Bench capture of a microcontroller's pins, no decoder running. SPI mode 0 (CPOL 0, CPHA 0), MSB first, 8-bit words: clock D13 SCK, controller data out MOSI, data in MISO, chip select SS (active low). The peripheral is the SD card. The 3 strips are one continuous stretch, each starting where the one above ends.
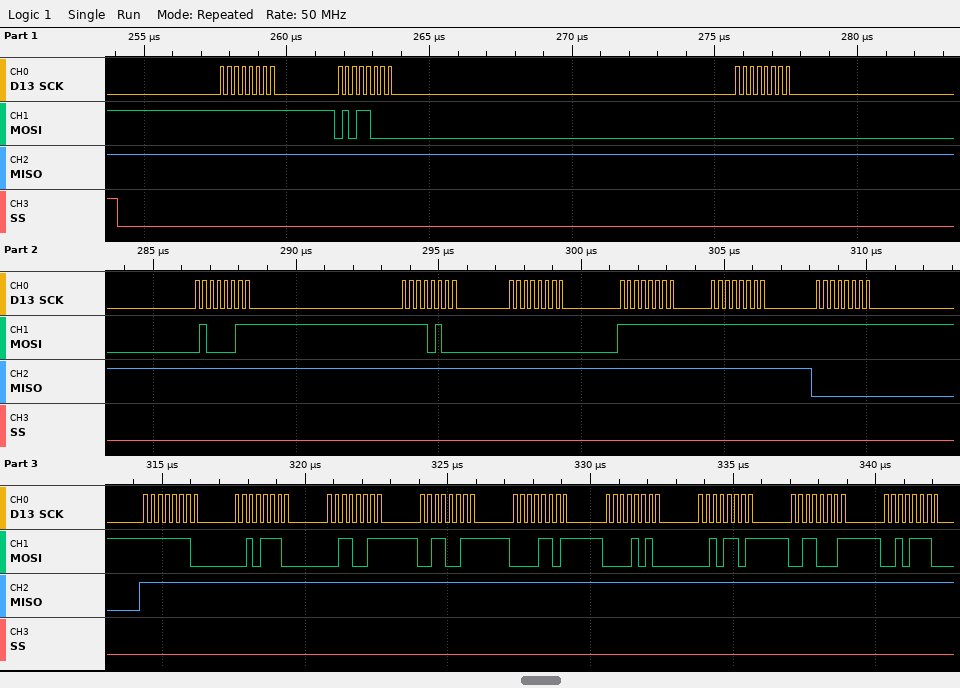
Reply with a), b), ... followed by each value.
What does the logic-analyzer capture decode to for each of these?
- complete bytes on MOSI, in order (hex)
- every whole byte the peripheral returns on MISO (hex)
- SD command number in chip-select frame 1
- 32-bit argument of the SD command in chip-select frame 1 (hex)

a) 0xFF 0x58 0x00 0x43 0xF4 0x00 0xFF 0xFF 0xFF 0xFE 0x2E 0x33 0x33 0x0D 0x0A 0x2D 0x31 0x2E
b) 0xFF 0xFF 0xFF 0xFF 0xFF 0xFF 0xFF 0xFF 0x00 0xFF 0xFF 0xFF 0xFF 0xFF 0xFF 0xFF 0xFF 0xFF
c) CMD24
d) 0x0043F400
